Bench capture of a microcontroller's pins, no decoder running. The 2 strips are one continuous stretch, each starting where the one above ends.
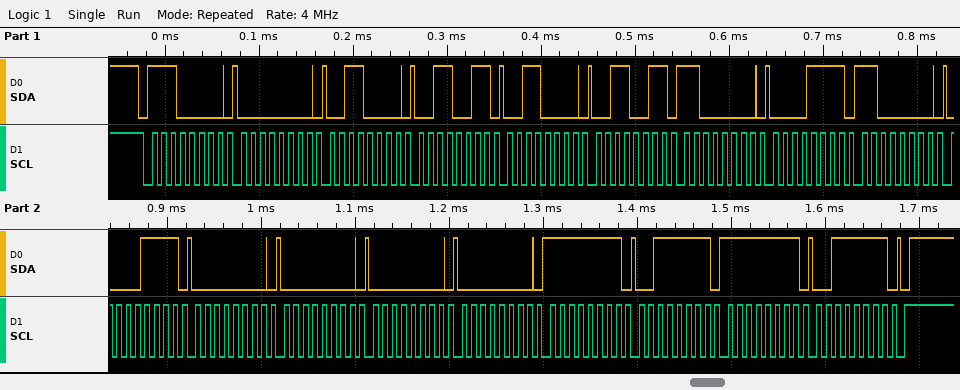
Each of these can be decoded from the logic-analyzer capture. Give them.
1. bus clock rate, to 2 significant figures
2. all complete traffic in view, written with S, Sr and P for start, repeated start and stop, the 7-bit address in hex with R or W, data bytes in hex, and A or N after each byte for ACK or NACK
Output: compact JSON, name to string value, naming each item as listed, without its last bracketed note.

{"bus clock rate, to 2 significant figures": "100 kHz", "all complete traffic in view, written with S, Sr and P for start, repeated start and stop, the 7-bit address in hex with R or W, data bytes in hex, and A or N after each byte for ACK or NACK": "S 70W A 00 A 30 A 33 A 30 A 33 A C0 A 0F A C0 A 0F A 00 A 00 A 00 A 00 A FF A 3F A FF A 3F A P"}
